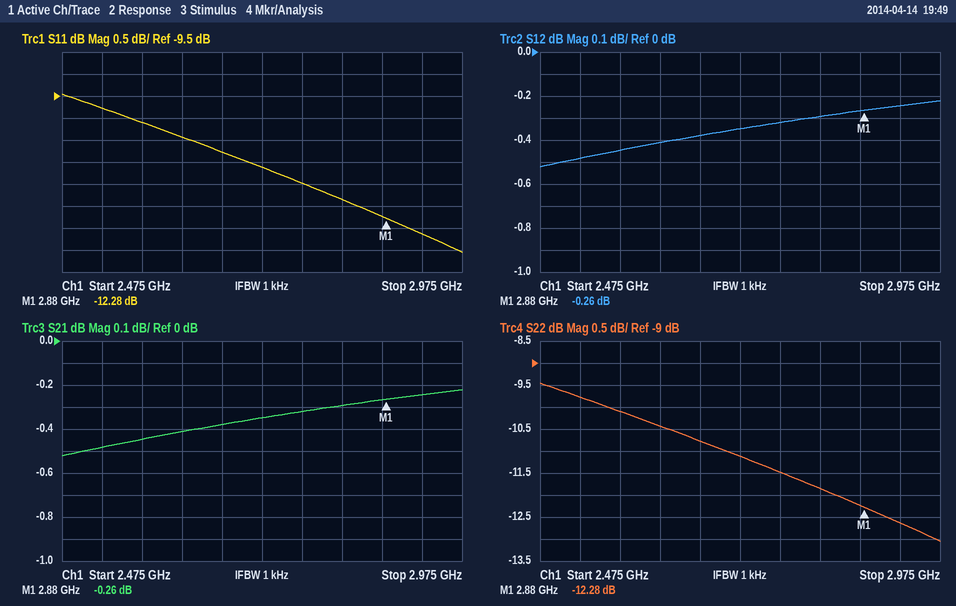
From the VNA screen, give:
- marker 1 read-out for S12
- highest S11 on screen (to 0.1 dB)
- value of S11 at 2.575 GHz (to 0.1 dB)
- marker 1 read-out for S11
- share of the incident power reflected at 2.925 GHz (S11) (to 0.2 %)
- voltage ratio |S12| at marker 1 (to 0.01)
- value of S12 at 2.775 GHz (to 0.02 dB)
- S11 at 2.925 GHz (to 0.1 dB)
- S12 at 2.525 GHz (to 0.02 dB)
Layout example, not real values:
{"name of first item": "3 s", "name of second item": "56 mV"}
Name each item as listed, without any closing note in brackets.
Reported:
{"marker 1 read-out for S12": "-0.26 dB", "highest S11 on screen": "-9.5 dB", "value of S11 at 2.575 GHz": "-10.1 dB", "marker 1 read-out for S11": "-12.28 dB", "share of the incident power reflected at 2.925 GHz (S11)": "5.4 %", "voltage ratio |S12| at marker 1": "0.97", "value of S12 at 2.775 GHz": "-0.32 dB", "S11 at 2.925 GHz": "-12.6 dB", "S12 at 2.525 GHz": "-0.48 dB"}
